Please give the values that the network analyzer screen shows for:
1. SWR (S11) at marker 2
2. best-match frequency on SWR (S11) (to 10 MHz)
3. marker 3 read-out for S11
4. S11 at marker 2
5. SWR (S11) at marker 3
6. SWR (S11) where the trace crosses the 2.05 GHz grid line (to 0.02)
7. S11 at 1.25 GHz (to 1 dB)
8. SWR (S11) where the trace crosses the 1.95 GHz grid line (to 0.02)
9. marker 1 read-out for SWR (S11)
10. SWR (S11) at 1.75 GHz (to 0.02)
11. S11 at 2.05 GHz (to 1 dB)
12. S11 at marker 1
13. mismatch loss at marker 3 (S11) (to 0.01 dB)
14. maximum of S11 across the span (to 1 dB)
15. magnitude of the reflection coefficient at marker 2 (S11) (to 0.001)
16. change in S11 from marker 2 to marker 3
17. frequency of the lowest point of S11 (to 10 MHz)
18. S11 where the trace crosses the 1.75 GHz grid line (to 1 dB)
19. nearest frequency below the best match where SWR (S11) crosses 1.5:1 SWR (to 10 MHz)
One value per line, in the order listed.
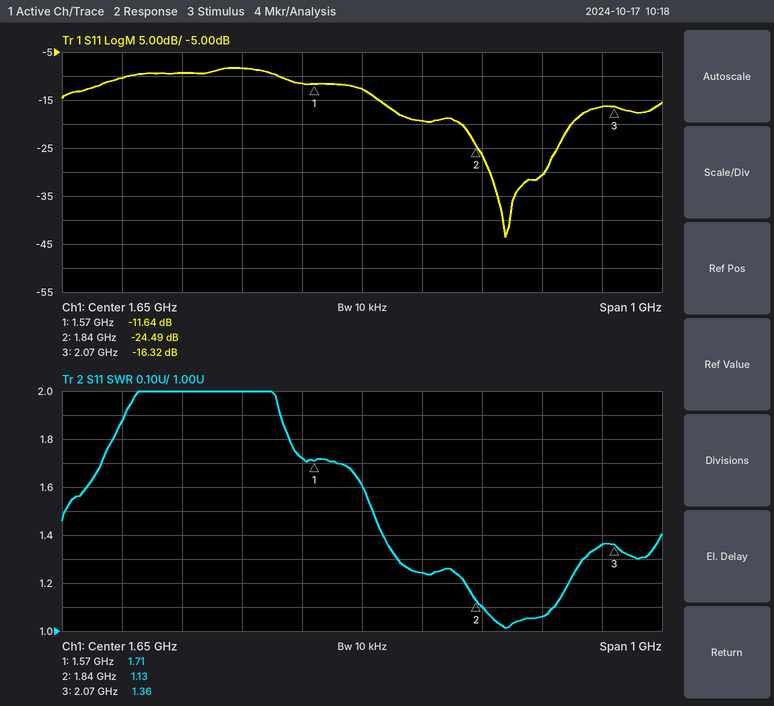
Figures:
1.13
1.89 GHz
-16.32 dB
-24.49 dB
1.36
1.36
-10 dB
1.06
1.71
1.24
-16 dB
-11.64 dB
0.10 dB
-8 dB
0.060
8.17 dB
1.89 GHz
-19 dB
1.67 GHz
